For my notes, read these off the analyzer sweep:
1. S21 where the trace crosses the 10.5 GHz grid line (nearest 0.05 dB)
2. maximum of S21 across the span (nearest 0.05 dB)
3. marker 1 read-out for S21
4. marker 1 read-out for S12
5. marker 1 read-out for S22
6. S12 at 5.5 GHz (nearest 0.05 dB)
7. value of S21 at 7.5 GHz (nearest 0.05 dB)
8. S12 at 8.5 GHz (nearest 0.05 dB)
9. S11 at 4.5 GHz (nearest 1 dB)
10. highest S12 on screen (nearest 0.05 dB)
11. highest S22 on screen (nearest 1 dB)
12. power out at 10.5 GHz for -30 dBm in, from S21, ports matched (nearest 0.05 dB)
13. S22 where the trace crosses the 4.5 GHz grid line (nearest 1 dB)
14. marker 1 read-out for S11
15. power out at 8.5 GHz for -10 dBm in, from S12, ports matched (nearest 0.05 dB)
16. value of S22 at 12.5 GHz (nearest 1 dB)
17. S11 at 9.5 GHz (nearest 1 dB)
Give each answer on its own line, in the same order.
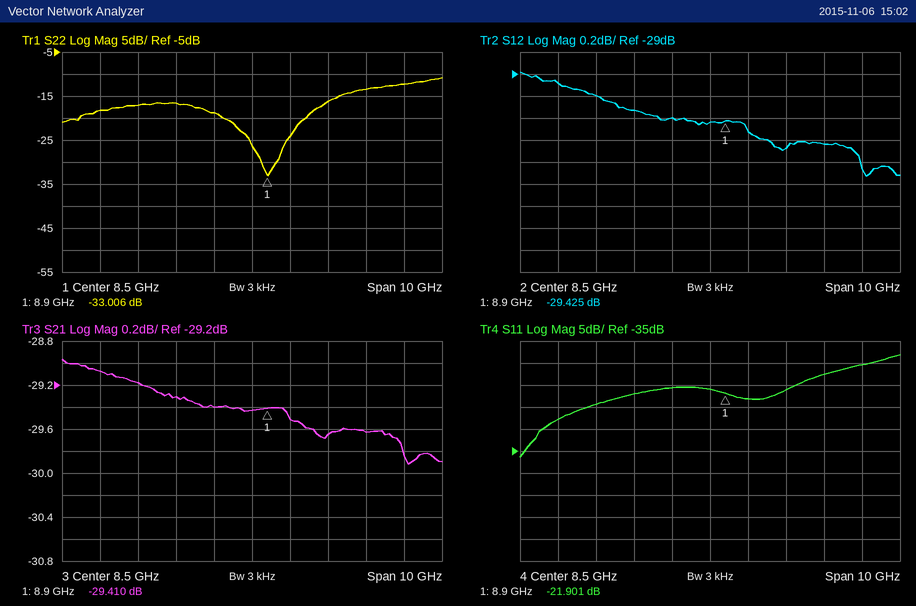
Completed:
-29.65 dB
-28.95 dB
-29.410 dB
-29.425 dB
-33.006 dB
-29.20 dB
-29.40 dB
-29.45 dB
-28 dB
-29.00 dB
-11 dB
-59.65 dBm
-18 dB
-21.901 dB
-39.45 dBm
-12 dB
-23 dB
